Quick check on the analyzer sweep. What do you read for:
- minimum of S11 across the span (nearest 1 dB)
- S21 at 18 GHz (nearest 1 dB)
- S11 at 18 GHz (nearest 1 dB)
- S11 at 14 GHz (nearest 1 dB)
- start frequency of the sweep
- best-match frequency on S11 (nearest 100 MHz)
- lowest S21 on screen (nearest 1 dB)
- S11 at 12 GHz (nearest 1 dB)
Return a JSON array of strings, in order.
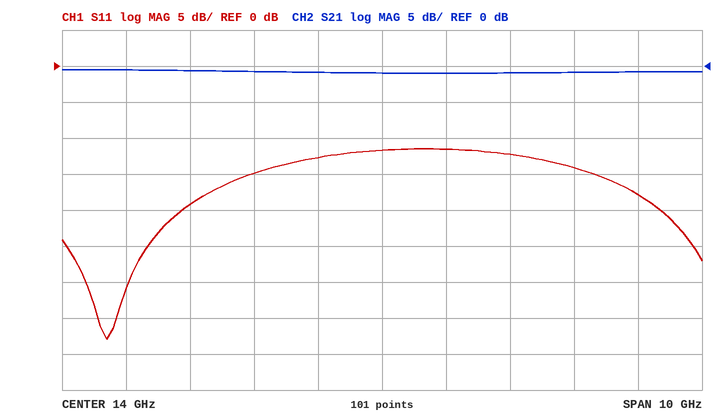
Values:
["-38 dB", "-1 dB", "-18 dB", "-12 dB", "9 GHz", "9.7 GHz", "-1 dB", "-15 dB"]
